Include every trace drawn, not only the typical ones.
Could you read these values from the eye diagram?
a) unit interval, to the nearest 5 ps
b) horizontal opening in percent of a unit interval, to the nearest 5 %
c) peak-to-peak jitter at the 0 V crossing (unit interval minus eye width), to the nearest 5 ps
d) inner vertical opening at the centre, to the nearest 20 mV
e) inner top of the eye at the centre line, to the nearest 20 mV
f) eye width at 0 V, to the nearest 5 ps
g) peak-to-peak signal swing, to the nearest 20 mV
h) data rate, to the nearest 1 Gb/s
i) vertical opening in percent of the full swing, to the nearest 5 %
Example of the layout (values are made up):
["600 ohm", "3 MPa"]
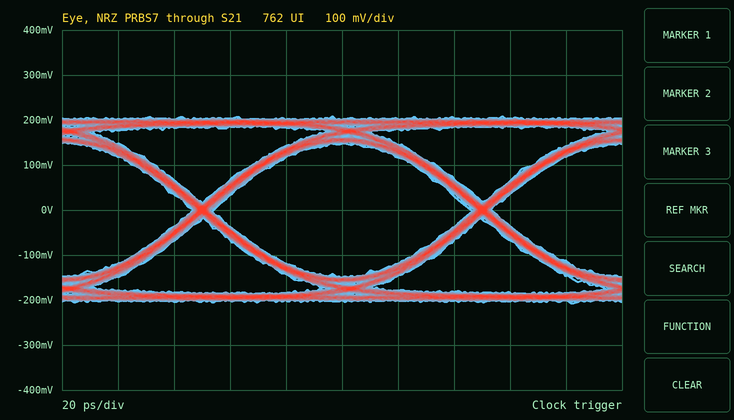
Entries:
["100 ps", "90 %", "10 ps", "300 mV", "140 mV", "90 ps", "420 mV", "10 Gb/s", "70 %"]
